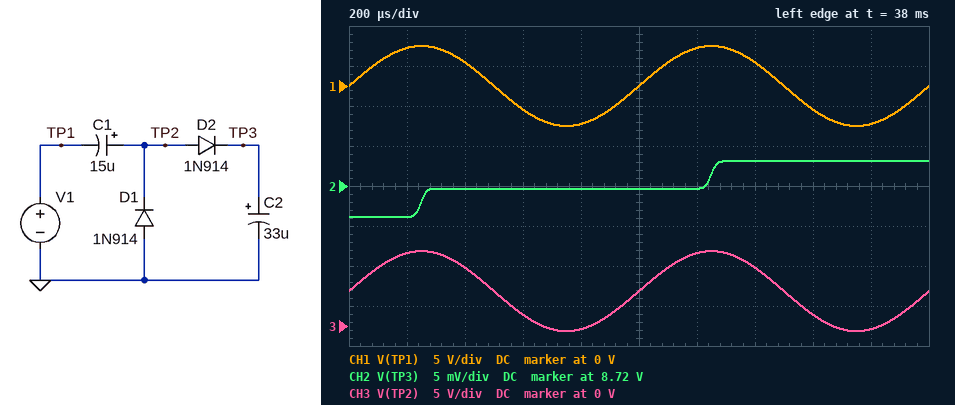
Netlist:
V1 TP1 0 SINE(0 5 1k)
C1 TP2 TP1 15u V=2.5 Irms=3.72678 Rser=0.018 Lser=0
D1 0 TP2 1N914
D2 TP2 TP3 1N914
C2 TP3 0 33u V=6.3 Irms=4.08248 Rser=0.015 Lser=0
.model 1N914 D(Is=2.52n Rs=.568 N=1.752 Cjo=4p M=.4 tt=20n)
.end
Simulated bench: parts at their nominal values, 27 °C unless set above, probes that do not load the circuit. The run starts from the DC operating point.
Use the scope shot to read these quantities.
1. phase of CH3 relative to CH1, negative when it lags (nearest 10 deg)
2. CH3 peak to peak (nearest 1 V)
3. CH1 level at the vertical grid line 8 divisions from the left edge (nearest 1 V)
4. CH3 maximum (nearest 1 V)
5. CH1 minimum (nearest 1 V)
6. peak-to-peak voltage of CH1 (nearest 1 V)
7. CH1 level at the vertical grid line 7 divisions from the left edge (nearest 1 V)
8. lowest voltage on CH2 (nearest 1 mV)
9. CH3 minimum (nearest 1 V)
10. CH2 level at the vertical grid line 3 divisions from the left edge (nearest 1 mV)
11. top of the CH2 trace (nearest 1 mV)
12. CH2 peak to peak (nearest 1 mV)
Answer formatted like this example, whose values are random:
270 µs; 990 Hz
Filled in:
0 deg; 10 V; -3 V; 9 V; -5 V; 10 V; 3 V; 8.716 V; -1 V; 8.720 V; 8.723 V; 7 mV
